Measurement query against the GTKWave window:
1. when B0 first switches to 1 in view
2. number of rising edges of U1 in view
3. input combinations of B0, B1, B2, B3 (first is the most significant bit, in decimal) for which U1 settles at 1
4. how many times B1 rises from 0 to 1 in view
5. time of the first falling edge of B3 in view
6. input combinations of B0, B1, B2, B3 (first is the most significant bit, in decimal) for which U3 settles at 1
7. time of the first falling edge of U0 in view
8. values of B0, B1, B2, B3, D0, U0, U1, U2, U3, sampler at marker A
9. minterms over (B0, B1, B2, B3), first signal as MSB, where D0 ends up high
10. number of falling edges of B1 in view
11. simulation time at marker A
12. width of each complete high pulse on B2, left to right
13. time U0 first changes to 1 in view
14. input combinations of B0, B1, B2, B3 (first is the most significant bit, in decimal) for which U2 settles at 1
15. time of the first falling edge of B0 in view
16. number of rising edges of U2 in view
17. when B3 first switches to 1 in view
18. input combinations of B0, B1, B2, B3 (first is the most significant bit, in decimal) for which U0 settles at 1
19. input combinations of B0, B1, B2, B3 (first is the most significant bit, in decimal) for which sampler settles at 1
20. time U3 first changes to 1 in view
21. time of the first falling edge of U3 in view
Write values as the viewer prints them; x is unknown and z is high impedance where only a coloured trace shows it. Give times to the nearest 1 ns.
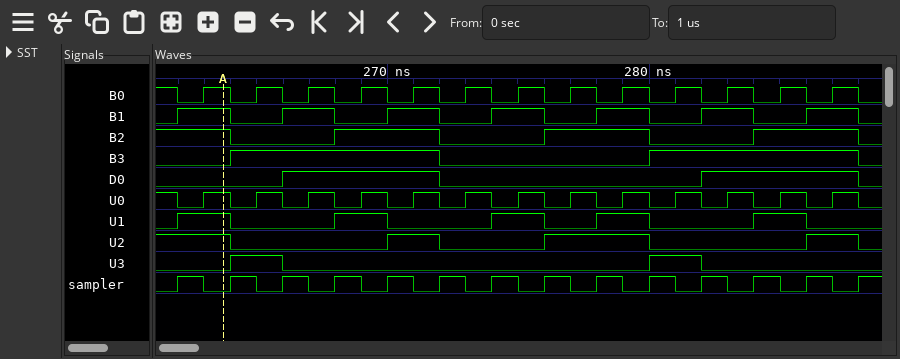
263 ns
5
3, 4, 6, 11, 12, 14
7
272 ns
1, 9
262 ns
B0=1, B1=1, B2=1, B3=0, D0=0, U0=1, U1=1, U2=1, U3=0, sampler=0
3, 5, 7, 11, 13, 15
7
264 ns
4 ns, 4 ns, 4 ns
263 ns
2, 6, 7, 10, 14, 15
262 ns
3
264 ns
8, 9, 10, 11, 12, 13, 14, 15
0, 1, 2, 3, 4, 5, 6, 7
264 ns
266 ns
